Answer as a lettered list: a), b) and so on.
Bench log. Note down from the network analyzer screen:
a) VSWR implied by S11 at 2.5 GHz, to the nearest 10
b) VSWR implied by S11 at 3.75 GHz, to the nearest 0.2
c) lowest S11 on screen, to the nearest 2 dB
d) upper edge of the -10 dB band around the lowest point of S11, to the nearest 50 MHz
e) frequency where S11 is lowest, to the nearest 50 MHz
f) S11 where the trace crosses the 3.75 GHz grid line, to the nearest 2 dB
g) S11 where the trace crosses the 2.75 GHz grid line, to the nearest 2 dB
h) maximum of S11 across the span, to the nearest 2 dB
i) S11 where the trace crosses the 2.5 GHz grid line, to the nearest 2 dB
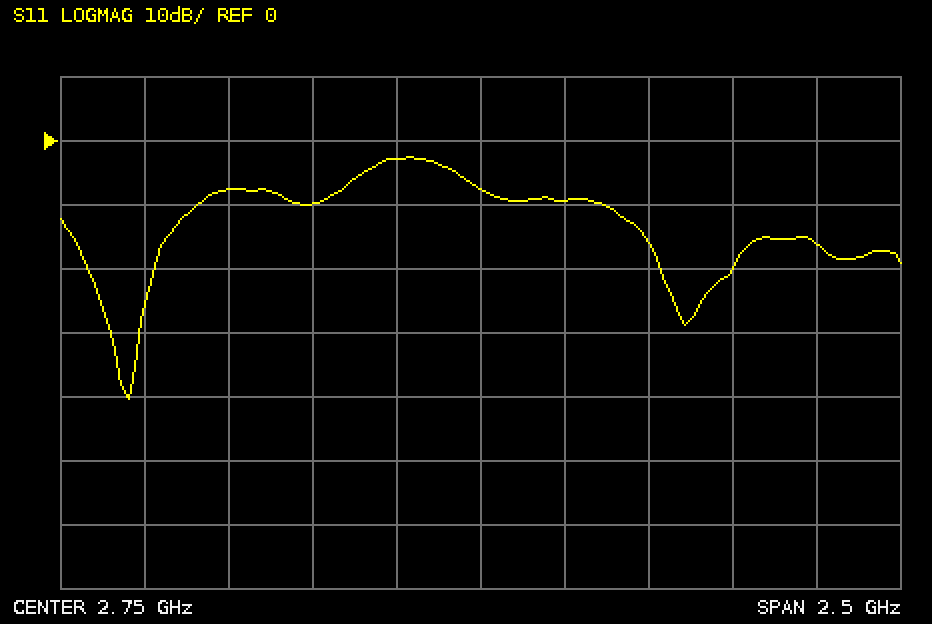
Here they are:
a) 10
b) 1.4
c) -40 dB
d) 1.90 GHz
e) 1.70 GHz
f) -16 dB
g) -8 dB
h) -2 dB
i) -2 dB
